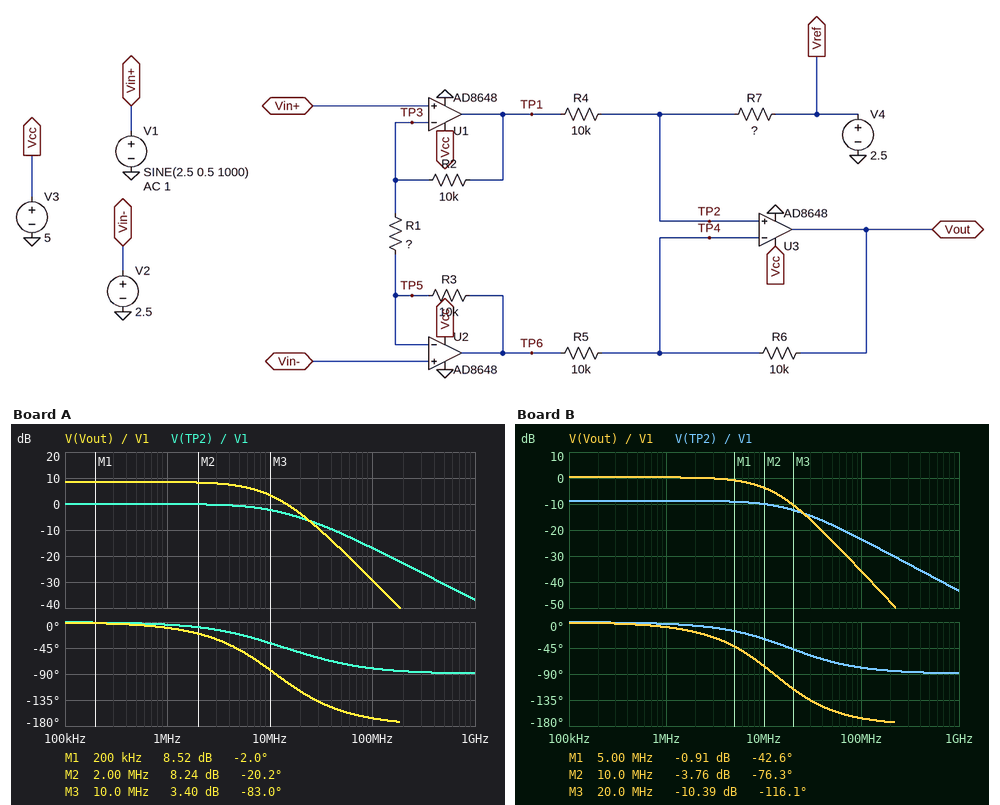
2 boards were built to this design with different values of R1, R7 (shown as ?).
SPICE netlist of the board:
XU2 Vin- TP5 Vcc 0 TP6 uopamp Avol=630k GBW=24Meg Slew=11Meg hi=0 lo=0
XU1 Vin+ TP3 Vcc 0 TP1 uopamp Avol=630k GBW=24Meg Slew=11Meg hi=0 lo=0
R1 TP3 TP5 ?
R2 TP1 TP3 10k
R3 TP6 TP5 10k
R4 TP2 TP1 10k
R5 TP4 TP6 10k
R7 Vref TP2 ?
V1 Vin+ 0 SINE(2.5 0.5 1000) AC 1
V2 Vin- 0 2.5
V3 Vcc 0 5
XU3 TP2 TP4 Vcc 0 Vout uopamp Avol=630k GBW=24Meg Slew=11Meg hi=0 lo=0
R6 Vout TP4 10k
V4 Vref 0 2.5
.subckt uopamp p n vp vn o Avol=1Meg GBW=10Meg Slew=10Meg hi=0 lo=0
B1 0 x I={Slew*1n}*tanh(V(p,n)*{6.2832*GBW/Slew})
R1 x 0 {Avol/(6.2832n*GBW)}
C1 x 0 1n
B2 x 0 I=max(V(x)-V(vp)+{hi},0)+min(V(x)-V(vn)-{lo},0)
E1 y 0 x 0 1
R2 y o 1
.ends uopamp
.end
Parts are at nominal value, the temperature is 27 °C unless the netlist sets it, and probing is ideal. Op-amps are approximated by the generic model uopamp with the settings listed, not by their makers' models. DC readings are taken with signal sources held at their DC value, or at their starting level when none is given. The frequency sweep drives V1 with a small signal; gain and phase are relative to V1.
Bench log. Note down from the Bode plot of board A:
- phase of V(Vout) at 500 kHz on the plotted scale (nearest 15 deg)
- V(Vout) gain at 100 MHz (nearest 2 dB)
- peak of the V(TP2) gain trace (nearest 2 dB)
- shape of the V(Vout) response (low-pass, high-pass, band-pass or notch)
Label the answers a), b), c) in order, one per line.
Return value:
a) 0 deg
b) -30 dB
c) 0 dB
d) low-pass
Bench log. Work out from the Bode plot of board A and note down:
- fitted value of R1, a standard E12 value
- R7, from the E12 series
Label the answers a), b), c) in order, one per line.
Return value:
a) 15 kΩ
b) 15 kΩ
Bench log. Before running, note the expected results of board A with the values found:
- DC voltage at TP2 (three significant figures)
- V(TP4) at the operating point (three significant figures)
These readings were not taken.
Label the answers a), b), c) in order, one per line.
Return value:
a) 2.50 V
b) 2.50 V
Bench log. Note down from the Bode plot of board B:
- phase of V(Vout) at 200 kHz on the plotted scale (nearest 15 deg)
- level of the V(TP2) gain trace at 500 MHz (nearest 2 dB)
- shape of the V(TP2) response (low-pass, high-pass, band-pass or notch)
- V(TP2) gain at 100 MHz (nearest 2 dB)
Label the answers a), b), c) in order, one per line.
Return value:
a) 0 deg
b) -38 dB
c) low-pass
d) -24 dB
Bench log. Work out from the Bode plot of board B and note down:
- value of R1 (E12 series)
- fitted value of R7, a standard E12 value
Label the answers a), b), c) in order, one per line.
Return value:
a) 33 kΩ
b) 3.9 kΩ
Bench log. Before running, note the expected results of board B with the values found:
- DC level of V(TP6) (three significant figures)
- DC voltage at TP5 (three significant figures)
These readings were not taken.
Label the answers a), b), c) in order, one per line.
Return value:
a) 2.50 V
b) 2.50 V
